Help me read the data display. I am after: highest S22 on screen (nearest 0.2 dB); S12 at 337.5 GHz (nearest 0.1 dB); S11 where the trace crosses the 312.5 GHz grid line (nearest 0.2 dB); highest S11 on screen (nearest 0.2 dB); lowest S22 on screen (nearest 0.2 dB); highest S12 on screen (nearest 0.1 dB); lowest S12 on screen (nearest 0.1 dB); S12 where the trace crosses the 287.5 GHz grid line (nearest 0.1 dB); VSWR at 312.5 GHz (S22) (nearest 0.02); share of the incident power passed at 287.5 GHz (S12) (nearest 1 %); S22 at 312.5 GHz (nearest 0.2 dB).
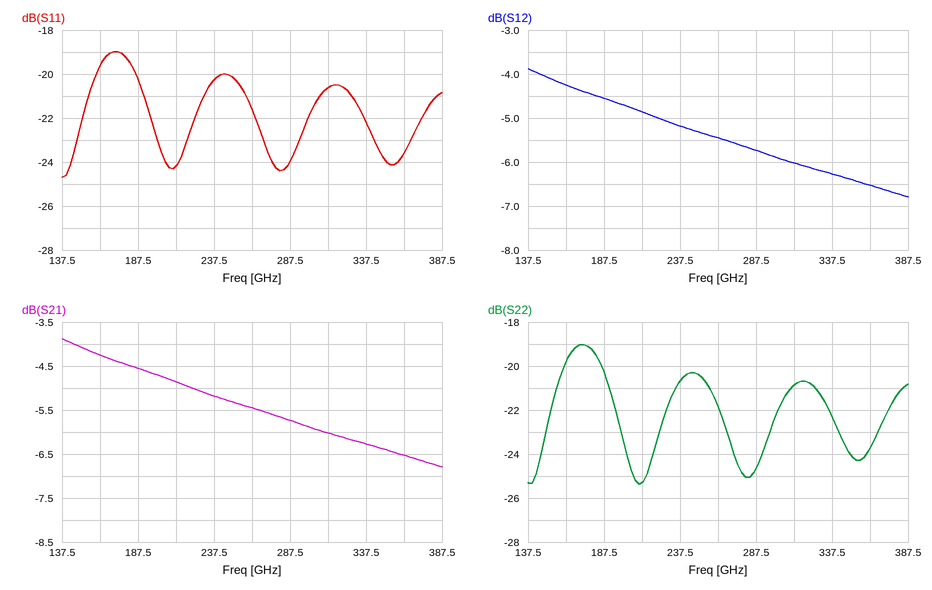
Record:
-19.0 dB
-6.3 dB
-20.6 dB
-19.0 dB
-25.4 dB
-3.9 dB
-6.8 dB
-5.7 dB
1.20
27 %
-20.8 dB
